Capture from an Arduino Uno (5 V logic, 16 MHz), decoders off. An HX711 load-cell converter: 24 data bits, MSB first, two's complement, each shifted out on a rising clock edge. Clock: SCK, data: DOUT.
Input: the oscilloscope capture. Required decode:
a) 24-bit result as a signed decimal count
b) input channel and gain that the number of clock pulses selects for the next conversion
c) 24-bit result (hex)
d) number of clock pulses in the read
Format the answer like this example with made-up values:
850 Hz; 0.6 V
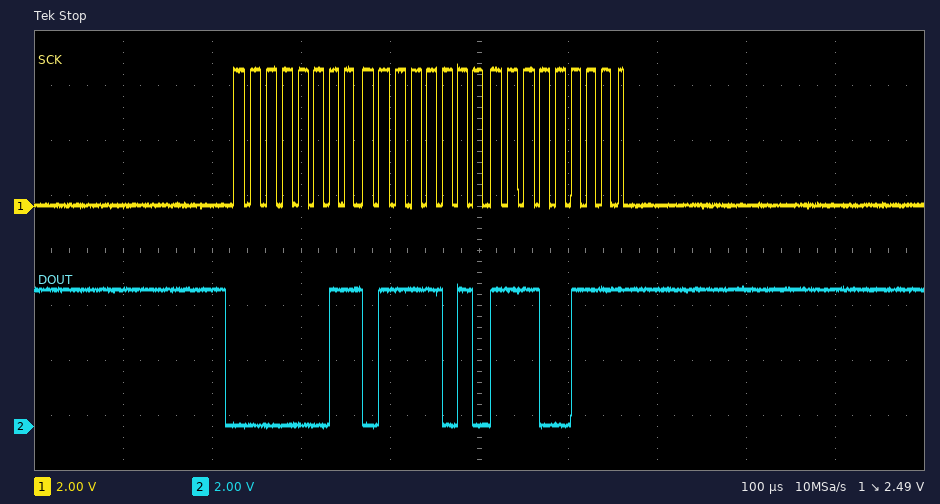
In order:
228071; channel A, gain 128; 0x037AE7; 25
